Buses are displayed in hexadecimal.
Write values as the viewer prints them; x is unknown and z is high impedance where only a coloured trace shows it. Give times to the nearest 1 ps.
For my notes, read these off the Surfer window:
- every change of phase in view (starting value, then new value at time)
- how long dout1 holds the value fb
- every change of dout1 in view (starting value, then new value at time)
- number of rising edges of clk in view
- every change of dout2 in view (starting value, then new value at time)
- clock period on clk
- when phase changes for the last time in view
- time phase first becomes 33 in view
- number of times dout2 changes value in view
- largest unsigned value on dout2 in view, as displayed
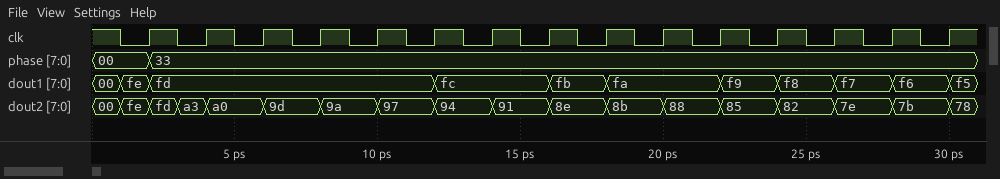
00, 33 at 2 ps
2 ps
00, fe at 1 ps, fd at 2 ps, fc at 12 ps, fb at 16 ps, fa at 18 ps, f9 at 22 ps, f8 at 24 ps, f7 at 26 ps, f6 at 28 ps, f5 at 30 ps
15
00, fe at 1 ps, fd at 2 ps, a3 at 3 ps, a0 at 4 ps, 9d at 6 ps, 9a at 8 ps, 97 at 10 ps, 94 at 12 ps, 91 at 14 ps, 8e at 16 ps, 8b at 18 ps, 88 at 20 ps, 85 at 22 ps, 82 at 24 ps, 7e at 26 ps, 7b at 28 ps, 78 at 30 ps
2 ps
2 ps
2 ps
17
fe
